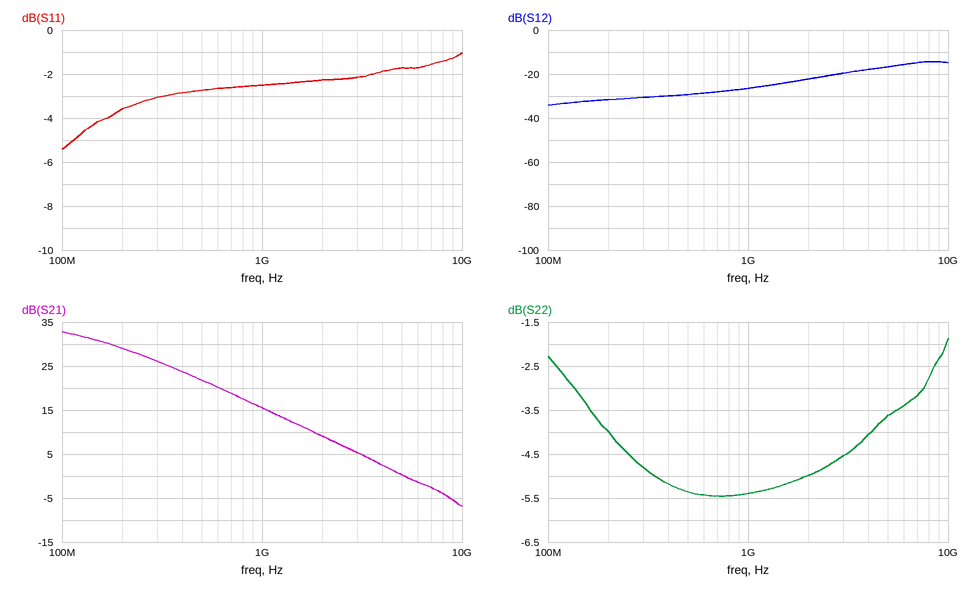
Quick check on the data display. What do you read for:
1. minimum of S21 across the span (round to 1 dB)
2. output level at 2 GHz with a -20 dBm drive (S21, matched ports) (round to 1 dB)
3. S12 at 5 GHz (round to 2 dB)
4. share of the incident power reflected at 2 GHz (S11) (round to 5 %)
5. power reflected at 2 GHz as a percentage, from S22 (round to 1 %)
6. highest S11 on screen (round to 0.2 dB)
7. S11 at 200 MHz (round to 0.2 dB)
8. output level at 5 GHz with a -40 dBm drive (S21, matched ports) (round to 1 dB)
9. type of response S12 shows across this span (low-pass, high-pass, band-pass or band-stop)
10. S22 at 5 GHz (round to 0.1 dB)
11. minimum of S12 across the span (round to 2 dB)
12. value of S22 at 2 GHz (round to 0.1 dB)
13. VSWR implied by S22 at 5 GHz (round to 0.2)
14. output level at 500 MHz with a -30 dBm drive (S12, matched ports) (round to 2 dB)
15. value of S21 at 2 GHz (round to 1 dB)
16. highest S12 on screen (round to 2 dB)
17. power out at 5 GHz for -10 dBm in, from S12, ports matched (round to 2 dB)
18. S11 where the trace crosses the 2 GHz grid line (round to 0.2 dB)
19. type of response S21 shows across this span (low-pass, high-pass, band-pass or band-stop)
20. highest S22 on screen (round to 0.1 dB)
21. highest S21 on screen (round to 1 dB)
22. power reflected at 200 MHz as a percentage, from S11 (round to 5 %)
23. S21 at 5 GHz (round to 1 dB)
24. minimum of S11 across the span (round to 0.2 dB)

-7 dB
-11 dBm
-16 dB
60 %
32 %
-1.0 dB
-3.6 dB
-40 dBm
high-pass
-3.6 dB
-34 dB
-5.0 dB
4.8
-60 dBm
9 dB
-14 dB
-26 dBm
-2.2 dB
low-pass
-1.9 dB
33 dB
45 %
0 dB
-5.4 dB
